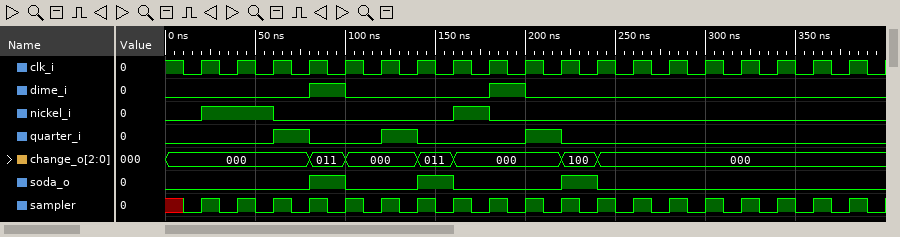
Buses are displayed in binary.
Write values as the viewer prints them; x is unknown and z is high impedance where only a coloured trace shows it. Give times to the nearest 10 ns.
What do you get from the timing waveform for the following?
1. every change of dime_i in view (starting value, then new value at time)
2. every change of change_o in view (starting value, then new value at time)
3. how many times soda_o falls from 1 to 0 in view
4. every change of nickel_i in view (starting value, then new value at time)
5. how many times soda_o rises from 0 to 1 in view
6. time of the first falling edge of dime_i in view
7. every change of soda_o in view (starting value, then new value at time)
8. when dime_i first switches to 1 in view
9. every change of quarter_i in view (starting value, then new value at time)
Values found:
0, 1 at 80 ns, 0 at 100 ns, 1 at 180 ns, 0 at 200 ns
000, 011 at 80 ns, 000 at 100 ns, 011 at 140 ns, 000 at 160 ns, 100 at 220 ns, 000 at 240 ns
3
0, 1 at 20 ns, 0 at 60 ns, 1 at 160 ns, 0 at 180 ns
3
100 ns
0, 1 at 80 ns, 0 at 100 ns, 1 at 140 ns, 0 at 160 ns, 1 at 220 ns, 0 at 240 ns
80 ns
0, 1 at 60 ns, 0 at 80 ns, 1 at 120 ns, 0 at 140 ns, 1 at 200 ns, 0 at 220 ns
